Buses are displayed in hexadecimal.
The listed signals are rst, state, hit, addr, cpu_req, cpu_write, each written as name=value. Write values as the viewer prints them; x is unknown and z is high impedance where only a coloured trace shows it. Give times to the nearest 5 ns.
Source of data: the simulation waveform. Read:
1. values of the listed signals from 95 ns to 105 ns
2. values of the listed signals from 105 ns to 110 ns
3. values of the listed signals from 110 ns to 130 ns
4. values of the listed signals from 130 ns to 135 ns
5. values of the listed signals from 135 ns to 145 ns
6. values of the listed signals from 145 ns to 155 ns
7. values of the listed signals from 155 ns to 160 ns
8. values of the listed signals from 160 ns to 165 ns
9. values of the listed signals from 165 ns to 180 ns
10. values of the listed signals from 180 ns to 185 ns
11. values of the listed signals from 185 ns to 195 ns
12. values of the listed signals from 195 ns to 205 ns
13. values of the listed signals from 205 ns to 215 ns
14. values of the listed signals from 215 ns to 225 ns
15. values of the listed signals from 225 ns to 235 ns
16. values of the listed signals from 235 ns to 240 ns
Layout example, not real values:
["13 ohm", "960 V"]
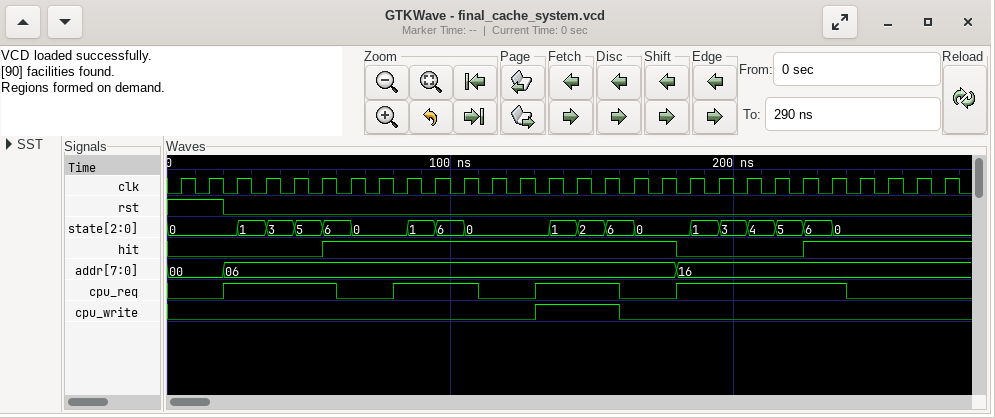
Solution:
["rst=0, state=6, hit=1, addr=06, cpu_req=1, cpu_write=0", "rst=0, state=0, hit=1, addr=06, cpu_req=1, cpu_write=0", "rst=0, state=0, hit=1, addr=06, cpu_req=0, cpu_write=0", "rst=0, state=0, hit=1, addr=06, cpu_req=1, cpu_write=1", "rst=0, state=1, hit=1, addr=06, cpu_req=1, cpu_write=1", "rst=0, state=2, hit=1, addr=06, cpu_req=1, cpu_write=1", "rst=0, state=6, hit=1, addr=06, cpu_req=1, cpu_write=1", "rst=0, state=6, hit=1, addr=06, cpu_req=0, cpu_write=0", "rst=0, state=0, hit=1, addr=06, cpu_req=0, cpu_write=0", "rst=0, state=0, hit=0, addr=16, cpu_req=1, cpu_write=0", "rst=0, state=1, hit=0, addr=16, cpu_req=1, cpu_write=0", "rst=0, state=3, hit=0, addr=16, cpu_req=1, cpu_write=0", "rst=0, state=4, hit=0, addr=16, cpu_req=1, cpu_write=0", "rst=0, state=5, hit=0, addr=16, cpu_req=1, cpu_write=0", "rst=0, state=6, hit=1, addr=16, cpu_req=1, cpu_write=0", "rst=0, state=0, hit=1, addr=16, cpu_req=1, cpu_write=0"]
